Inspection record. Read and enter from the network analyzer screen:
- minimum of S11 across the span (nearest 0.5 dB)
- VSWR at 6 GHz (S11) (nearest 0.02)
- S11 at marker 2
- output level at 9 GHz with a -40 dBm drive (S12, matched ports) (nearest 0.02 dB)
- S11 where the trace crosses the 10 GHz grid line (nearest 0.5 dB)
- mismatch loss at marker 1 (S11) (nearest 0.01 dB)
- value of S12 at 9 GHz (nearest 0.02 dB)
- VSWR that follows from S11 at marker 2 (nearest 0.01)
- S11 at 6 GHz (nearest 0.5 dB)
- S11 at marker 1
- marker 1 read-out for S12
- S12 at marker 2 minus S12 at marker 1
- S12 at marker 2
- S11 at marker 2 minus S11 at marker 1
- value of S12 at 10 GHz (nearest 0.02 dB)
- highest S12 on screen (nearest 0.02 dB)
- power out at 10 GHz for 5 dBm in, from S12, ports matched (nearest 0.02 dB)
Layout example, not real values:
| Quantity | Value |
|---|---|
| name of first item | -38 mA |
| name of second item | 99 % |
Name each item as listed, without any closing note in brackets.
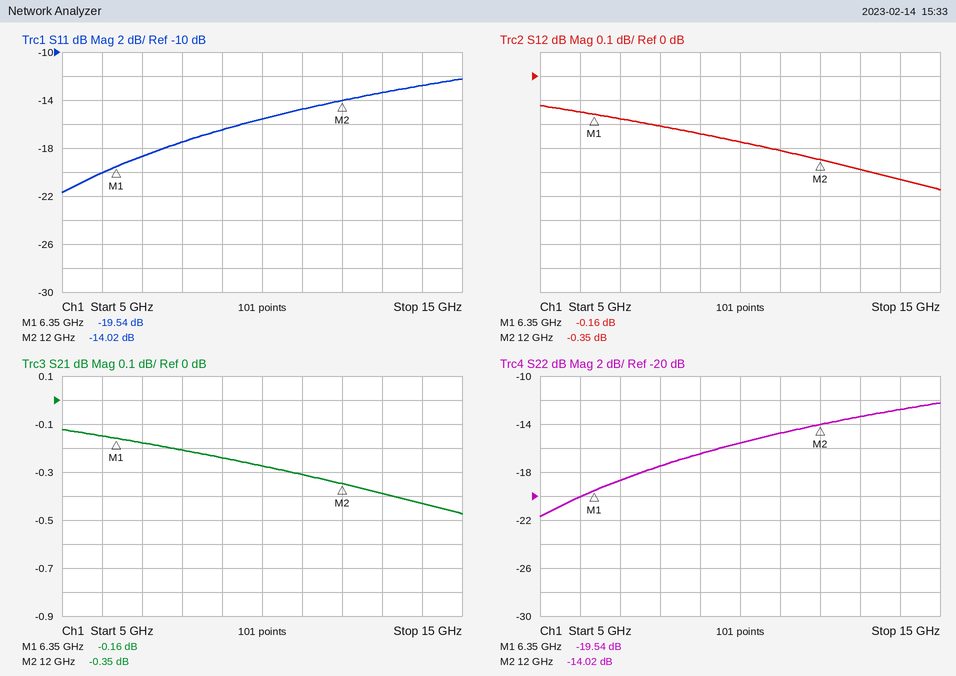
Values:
| Quantity | Value |
|---|---|
| minimum of S11 across the span | -21.5 dB |
| VSWR at 6 GHz (S11) | 1.22 |
| S11 at marker 2 | -14.02 dB |
| output level at 9 GHz with a -40 dBm drive (S12, matched ports) | -40.24 dBm |
| S11 where the trace crosses the 10 GHz grid line | -15.5 dB |
| mismatch loss at marker 1 (S11) | 0.05 dB |
| value of S12 at 9 GHz | -0.24 dB |
| VSWR that follows from S11 at marker 2 | 1.50 |
| S11 at 6 GHz | -20.0 dB |
| S11 at marker 1 | -19.54 dB |
| marker 1 read-out for S12 | -0.16 dB |
| S12 at marker 2 minus S12 at marker 1 | -0.19 dB |
| S12 at marker 2 | -0.35 dB |
| S11 at marker 2 minus S11 at marker 1 | 5.52 dB |
| value of S12 at 10 GHz | -0.28 dB |
| highest S12 on screen | -0.12 dB |
| power out at 10 GHz for 5 dBm in, from S12, ports matched | 4.72 dBm |
